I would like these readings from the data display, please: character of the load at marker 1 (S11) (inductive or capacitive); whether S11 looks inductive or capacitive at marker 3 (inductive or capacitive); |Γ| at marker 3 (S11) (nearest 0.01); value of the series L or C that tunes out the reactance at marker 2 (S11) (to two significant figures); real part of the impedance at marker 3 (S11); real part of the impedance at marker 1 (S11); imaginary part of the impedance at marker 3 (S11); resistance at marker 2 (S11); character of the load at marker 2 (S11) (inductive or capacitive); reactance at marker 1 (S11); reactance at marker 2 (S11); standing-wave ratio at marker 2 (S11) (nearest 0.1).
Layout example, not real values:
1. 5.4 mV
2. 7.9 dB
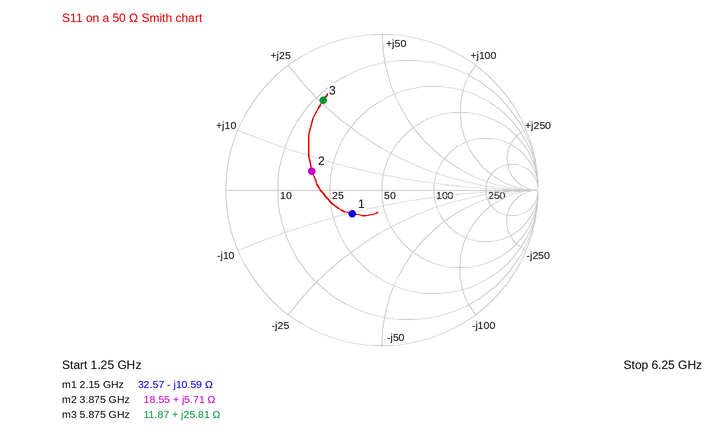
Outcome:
1. capacitive
2. inductive
3. 0.69
4. 7.2 pF
5. 11.87 Ω
6. 32.57 Ω
7. +25.81 Ω
8. 18.55 Ω
9. inductive
10. -10.59 Ω
11. +5.71 Ω
12. 2.7
